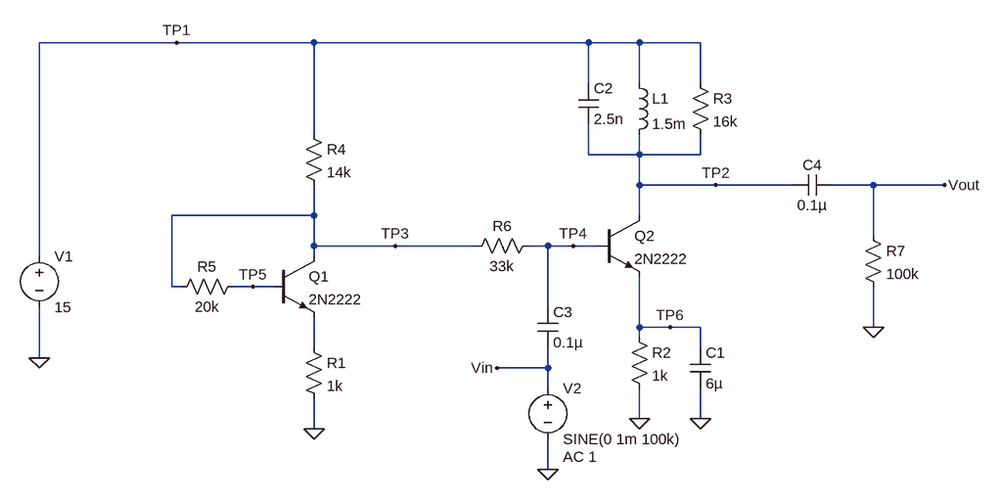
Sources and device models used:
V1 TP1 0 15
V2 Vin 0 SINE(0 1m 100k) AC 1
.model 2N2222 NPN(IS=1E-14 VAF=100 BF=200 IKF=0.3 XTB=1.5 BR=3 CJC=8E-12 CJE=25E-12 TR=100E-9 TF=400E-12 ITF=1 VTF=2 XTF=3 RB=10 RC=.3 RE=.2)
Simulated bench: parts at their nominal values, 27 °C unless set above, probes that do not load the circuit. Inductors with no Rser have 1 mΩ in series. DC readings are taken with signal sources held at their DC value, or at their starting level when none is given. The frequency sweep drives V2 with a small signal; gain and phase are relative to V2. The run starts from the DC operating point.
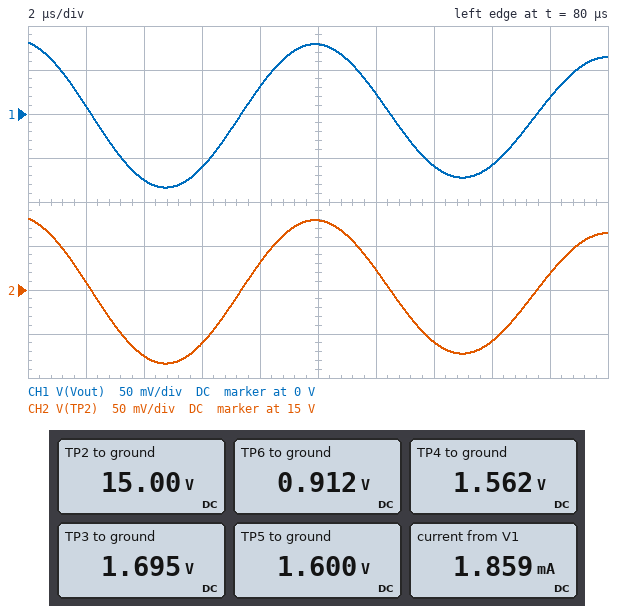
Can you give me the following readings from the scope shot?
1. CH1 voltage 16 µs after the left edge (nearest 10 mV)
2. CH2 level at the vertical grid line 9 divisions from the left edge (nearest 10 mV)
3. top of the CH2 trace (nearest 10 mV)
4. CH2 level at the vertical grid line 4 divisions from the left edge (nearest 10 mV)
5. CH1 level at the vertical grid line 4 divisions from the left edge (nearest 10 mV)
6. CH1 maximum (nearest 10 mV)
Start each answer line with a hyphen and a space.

- -60 mV
- 15.02 V
- 15.08 V
- 15.03 V
- 30 mV
- 80 mV
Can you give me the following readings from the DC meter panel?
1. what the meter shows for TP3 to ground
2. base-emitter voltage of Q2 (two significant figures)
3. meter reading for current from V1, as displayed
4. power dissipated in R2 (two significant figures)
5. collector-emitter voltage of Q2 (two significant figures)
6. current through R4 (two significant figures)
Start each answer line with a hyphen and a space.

- 1.695 V
- 650 mV
- 1.859 mA
- 830 µW
- 14 V
- 950 µA
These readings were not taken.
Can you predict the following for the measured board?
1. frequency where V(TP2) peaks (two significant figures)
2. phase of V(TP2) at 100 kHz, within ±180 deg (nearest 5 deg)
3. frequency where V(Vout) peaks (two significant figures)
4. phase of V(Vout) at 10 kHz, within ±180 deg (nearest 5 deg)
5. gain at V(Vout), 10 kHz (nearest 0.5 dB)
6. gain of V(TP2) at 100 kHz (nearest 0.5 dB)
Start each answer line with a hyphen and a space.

- 82 kHz
- 100 deg
- 82 kHz
- -85 deg
- 10.5 dB
- 36.5 dB
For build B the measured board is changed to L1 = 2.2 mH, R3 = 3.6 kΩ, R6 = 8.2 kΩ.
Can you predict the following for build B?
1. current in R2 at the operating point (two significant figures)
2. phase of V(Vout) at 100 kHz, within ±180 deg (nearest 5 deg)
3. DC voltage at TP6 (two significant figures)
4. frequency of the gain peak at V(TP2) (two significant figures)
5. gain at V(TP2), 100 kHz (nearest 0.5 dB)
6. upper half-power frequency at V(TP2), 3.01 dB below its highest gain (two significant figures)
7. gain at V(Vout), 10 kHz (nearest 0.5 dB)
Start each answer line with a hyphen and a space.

- 1.0 mA
- 110 deg
- 1.0 V
- 68 kHz
- 32.5 dB
- 78 kHz
- 14.5 dB
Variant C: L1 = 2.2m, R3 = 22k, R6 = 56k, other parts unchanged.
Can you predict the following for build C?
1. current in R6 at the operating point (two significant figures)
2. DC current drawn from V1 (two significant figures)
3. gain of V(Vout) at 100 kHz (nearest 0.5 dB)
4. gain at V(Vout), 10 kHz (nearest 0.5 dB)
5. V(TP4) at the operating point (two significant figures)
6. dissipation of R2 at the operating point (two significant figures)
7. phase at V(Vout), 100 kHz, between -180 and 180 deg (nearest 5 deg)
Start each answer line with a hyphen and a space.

- 3.7 µA
- 1.8 mA
- 31.5 dB
- 13.0 dB
- 1.5 V
- 710 µW
- 95 deg
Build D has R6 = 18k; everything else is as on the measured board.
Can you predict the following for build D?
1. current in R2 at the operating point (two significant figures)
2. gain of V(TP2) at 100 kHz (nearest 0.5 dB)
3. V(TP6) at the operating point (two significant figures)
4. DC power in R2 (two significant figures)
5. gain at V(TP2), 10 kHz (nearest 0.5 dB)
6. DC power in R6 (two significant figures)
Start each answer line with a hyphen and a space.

- 970 µA
- 37.0 dB
- 970 mV
- 930 µW
- 11.0 dB
- 330 nW
